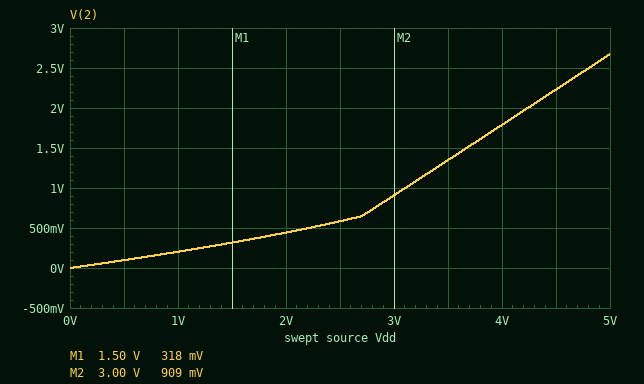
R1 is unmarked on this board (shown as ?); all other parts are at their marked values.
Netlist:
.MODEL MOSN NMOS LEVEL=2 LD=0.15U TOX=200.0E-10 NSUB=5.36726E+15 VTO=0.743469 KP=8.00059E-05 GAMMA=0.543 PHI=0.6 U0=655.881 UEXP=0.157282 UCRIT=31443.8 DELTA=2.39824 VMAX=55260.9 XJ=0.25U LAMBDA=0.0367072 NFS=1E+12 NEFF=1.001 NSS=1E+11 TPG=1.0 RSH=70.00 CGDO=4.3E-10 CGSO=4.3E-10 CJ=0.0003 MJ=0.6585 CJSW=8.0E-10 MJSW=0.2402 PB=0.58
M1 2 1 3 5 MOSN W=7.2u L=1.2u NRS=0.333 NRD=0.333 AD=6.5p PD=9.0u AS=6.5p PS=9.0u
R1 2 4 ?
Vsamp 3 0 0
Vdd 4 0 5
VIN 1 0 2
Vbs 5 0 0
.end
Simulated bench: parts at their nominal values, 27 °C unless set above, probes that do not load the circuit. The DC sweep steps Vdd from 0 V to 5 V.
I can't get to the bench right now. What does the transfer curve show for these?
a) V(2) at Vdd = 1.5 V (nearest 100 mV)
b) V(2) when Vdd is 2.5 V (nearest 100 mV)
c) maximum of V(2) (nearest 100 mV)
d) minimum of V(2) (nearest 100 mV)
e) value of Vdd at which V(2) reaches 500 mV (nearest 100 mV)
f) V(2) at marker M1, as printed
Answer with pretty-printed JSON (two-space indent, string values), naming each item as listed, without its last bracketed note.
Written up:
{
  "V(2) at Vdd = 1.5 V": "300 mV",
  "V(2) when Vdd is 2.5 V": "600 mV",
  "maximum of V(2)": "2.7 V",
  "minimum of V(2)": "0 V",
  "value of Vdd at which V(2) reaches 500 mV": "2.2 V",
  "V(2) at marker M1, as printed": "318 mV"
}
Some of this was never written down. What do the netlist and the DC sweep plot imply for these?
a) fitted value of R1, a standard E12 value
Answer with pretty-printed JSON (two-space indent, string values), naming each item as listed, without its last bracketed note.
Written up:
{
  "fitted value of R1, a standard E12 value": "6.8 kΩ"
}
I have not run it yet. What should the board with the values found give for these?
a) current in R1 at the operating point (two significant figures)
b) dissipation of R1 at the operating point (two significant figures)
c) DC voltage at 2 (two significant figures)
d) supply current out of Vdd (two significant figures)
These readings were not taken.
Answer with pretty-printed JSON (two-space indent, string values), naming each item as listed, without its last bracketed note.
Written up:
{
  "current in R1 at the operating point": "340 µA",
  "dissipation of R1 at the operating point": "800 µW",
  "DC voltage at 2": "2.7 V",
  "supply current out of Vdd": "340 µA"
}
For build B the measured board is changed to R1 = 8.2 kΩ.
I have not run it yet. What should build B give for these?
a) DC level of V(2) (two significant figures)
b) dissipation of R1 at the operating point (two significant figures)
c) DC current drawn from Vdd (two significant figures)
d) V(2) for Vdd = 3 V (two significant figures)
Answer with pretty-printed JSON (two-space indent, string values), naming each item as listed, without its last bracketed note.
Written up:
{
  "DC level of V(2)": "2.3 V",
  "dissipation of R1 at the operating point": "920 µW",
  "DC current drawn from Vdd": "330 µA",
  "V(2) for Vdd = 3 V": "610 mV"
}
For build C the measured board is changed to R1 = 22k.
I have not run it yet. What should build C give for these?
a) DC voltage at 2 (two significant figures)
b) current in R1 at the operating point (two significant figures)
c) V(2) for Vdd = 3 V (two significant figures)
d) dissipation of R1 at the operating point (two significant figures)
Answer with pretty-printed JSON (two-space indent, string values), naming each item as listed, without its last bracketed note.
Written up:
{
  "DC voltage at 2": "400 mV",
  "current in R1 at the operating point": "210 µA",
  "V(2) for Vdd = 3 V": "220 mV",
  "dissipation of R1 at the operating point": "960 µW"
}
